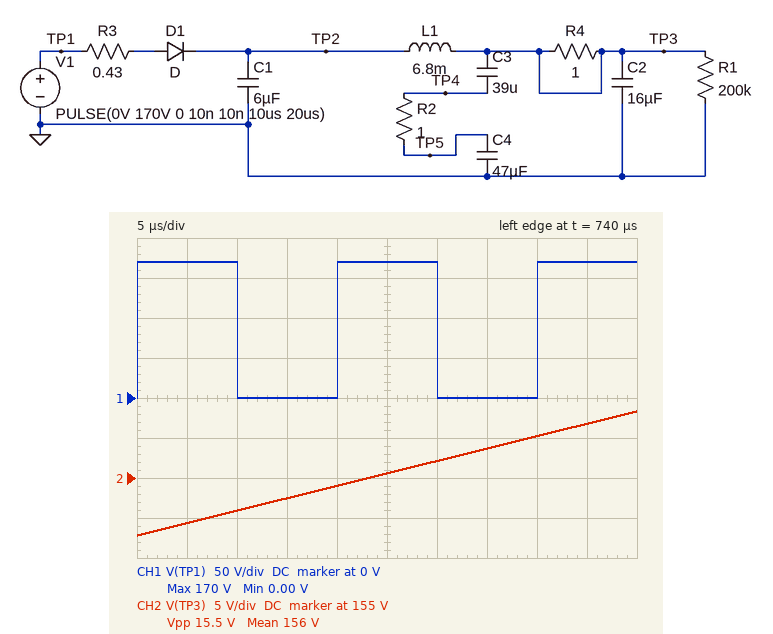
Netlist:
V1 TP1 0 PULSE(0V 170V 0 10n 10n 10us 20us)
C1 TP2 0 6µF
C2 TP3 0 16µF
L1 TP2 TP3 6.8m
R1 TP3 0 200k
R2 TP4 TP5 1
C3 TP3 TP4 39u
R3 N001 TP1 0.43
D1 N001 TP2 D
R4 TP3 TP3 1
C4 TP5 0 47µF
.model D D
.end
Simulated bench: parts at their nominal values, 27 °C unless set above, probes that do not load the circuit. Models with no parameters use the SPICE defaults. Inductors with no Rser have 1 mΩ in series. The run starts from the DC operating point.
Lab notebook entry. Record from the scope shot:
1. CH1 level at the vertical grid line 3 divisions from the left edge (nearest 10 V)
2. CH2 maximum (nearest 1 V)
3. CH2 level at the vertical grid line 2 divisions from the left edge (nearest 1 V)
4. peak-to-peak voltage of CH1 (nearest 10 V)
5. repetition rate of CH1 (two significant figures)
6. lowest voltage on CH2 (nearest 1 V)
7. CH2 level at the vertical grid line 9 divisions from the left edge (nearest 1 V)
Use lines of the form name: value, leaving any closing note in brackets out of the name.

CH1 level at the vertical grid line 3 divisions from the left edge: 0 V
CH2 maximum: 163 V
CH2 level at the vertical grid line 2 divisions from the left edge: 151 V
peak-to-peak voltage of CH1: 170 V
repetition rate of CH1: 50 kHz
lowest voltage on CH2: 148 V
CH2 level at the vertical grid line 9 divisions from the left edge: 162 V
